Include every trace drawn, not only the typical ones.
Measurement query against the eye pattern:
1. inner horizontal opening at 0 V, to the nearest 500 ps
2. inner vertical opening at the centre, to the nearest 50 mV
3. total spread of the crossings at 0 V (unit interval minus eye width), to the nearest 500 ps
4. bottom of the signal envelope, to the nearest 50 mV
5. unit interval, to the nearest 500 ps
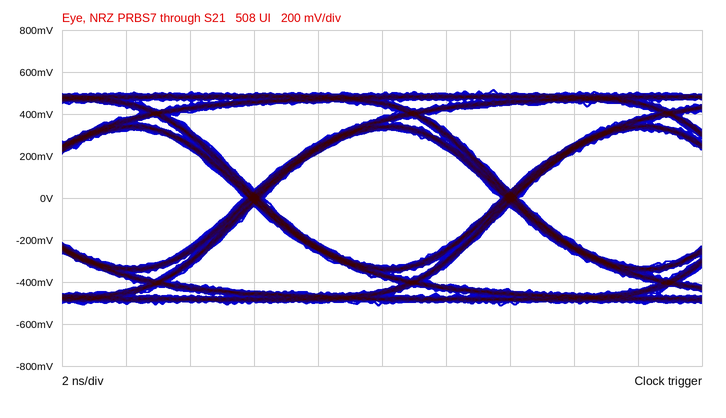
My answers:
7.5 ns
650 mV
500 ps
-500 mV
8.0 ns
